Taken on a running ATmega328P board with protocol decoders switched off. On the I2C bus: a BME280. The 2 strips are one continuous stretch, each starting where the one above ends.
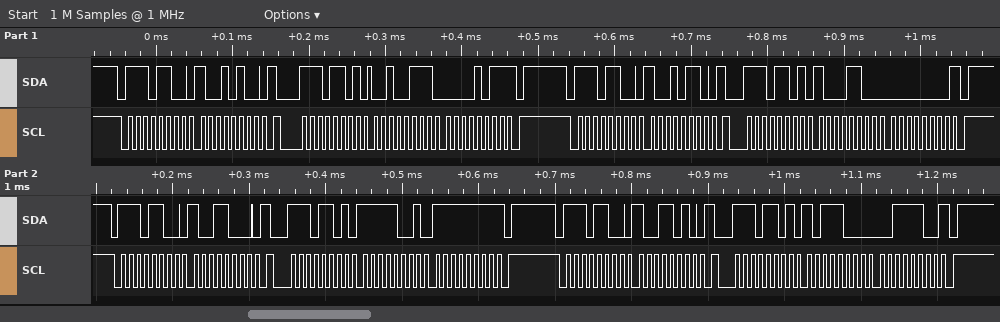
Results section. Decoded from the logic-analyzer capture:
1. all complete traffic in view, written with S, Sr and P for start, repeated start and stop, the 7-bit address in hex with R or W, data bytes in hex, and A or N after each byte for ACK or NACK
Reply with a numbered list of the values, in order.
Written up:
1. S 76W A 94 A Sr 76R A 27 A 0B N P S 76W A 96 A Sr 76R A 8C A 00 N P S 76W A 98 A Sr 76R A F9 A FF N P S 76W A 9A A Sr 76R A B8 A 3C N P
